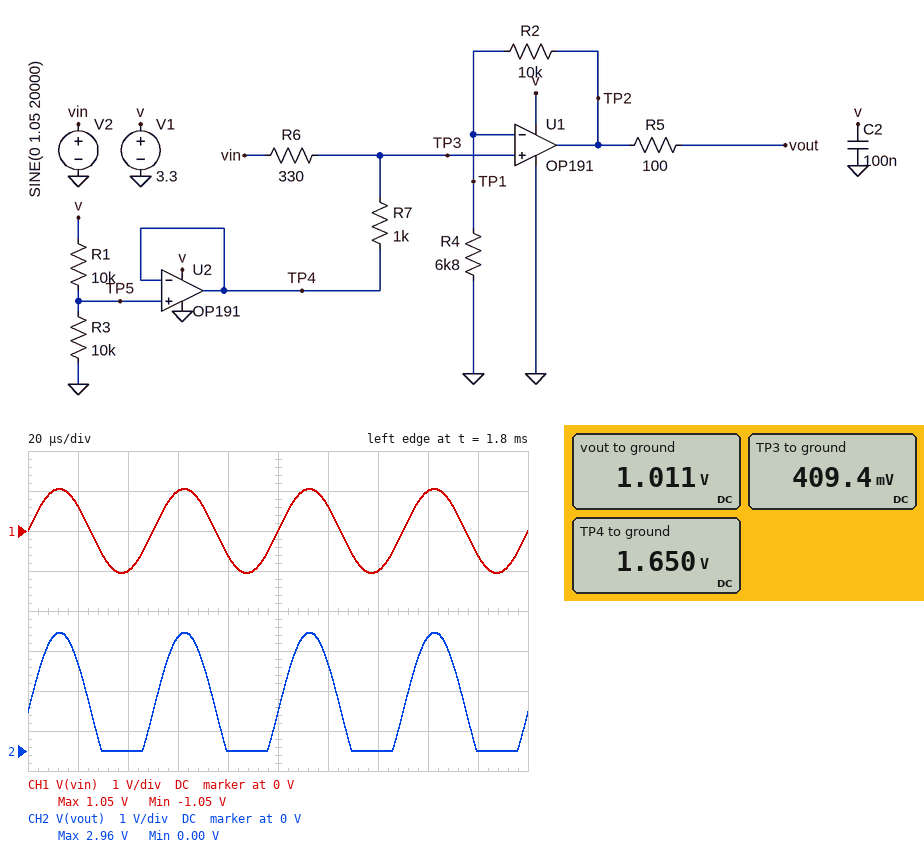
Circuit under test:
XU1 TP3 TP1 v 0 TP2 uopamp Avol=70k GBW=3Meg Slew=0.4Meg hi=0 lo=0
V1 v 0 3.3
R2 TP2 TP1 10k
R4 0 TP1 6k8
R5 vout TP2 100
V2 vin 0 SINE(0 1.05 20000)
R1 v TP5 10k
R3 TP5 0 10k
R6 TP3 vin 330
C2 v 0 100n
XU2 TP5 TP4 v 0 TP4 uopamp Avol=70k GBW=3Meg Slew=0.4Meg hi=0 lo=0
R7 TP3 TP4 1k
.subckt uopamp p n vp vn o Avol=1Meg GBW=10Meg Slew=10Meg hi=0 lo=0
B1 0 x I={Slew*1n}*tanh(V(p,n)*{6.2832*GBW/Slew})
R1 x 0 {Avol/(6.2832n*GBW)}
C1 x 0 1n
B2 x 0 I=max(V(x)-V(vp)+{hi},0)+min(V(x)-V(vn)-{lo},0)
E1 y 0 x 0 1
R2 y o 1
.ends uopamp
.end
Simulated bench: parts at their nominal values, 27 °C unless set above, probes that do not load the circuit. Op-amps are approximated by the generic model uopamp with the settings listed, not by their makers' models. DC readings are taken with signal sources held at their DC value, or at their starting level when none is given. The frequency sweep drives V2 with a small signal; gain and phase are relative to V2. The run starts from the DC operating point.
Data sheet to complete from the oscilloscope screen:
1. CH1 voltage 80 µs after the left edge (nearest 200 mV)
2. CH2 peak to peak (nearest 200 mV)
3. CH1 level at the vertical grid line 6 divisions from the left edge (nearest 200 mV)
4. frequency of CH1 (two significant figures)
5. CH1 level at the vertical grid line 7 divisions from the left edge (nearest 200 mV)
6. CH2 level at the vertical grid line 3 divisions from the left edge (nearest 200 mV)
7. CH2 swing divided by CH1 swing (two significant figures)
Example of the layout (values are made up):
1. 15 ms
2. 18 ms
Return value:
1. -600 mV
2. 3.0 V
3. 600 mV
4. 20 kHz
5. -1.0 V
6. 2.8 V
7. 1.4
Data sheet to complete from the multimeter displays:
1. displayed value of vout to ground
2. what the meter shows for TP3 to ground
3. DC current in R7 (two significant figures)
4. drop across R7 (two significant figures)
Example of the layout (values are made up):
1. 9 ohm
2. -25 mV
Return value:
1. 1.011 V
2. 409.4 mV
3. 1.2 mA
4. 1.2 V
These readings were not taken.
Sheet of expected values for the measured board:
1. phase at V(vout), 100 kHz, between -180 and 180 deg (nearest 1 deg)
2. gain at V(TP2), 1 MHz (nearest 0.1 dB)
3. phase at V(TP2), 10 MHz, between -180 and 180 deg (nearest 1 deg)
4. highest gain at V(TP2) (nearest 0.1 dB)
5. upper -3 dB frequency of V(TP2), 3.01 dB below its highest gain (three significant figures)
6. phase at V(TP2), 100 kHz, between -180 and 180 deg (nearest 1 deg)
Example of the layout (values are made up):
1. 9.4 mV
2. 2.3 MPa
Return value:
1. -5 deg
2. 3.1 dB
3. -83 deg
4. 5.4 dB
5. 1.21 MHz
6. -5 deg
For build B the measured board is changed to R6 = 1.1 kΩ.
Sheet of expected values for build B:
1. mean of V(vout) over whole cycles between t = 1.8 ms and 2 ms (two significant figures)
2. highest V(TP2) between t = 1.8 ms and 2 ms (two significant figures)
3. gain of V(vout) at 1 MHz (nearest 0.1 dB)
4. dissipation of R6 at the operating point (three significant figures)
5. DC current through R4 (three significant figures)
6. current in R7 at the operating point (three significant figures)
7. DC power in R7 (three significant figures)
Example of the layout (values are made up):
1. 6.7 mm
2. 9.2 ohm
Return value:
1. 2.1 V
2. 3.3 V
3. -0.8 dB
4. 679 µW
5. 127 µA
6. 786 µA
7. 617 µW
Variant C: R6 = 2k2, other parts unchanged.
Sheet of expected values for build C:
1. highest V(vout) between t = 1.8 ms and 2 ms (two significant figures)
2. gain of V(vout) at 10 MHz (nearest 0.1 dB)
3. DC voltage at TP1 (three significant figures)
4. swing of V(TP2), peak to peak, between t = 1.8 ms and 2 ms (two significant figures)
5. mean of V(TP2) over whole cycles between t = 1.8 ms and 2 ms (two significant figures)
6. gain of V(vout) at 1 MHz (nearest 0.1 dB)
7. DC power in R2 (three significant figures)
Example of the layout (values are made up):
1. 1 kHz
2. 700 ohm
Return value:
1. 3.3 V
2. -20.6 dB
3. 1.13 V
4. 1.3 V
5. 2.7 V
6. -4.5 dB
7. 278 µW
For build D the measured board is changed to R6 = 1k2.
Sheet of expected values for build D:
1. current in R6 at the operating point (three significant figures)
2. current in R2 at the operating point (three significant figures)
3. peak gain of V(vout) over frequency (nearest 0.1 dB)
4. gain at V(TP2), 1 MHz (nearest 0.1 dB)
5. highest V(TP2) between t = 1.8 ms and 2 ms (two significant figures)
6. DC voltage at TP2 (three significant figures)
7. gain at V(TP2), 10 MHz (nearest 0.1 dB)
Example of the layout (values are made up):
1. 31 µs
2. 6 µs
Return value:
1. 750 µA
2. 132 µA
3. 1.0 dB
4. -1.2 dB
5. 3.3 V
6. 2.22 V
7. -17.4 dB
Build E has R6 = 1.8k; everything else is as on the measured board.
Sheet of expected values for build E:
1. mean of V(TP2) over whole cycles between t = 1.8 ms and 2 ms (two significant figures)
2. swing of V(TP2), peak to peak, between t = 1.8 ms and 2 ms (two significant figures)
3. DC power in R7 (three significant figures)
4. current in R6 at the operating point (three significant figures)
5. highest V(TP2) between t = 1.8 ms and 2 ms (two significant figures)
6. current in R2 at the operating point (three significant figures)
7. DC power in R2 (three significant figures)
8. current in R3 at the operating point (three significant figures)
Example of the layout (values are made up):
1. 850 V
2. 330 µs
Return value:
1. 2.6 V
2. 1.6 V
3. 347 µW
4. 589 µA
5. 3.3 V
6. 156 µA
7. 243 µW
8. 165 µA
